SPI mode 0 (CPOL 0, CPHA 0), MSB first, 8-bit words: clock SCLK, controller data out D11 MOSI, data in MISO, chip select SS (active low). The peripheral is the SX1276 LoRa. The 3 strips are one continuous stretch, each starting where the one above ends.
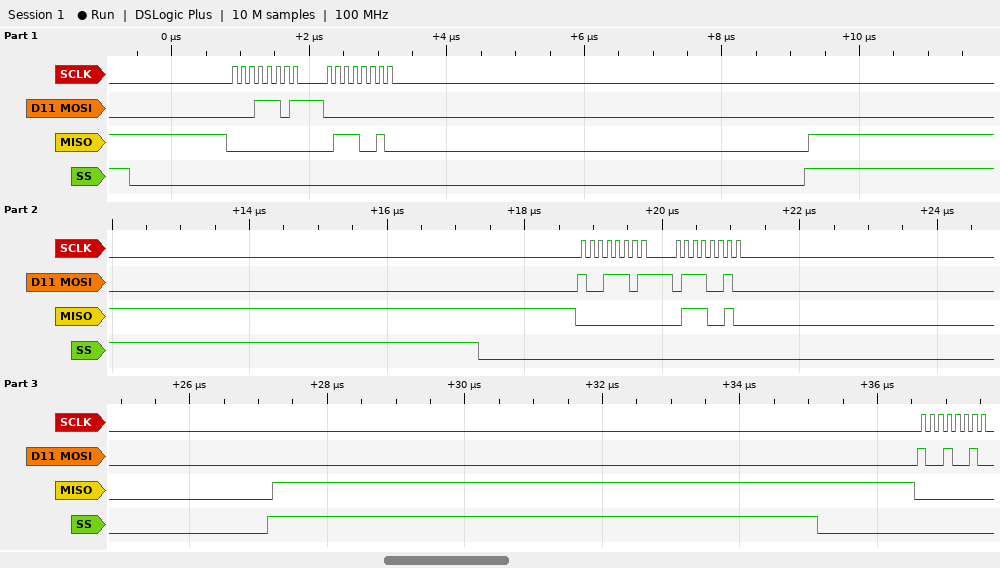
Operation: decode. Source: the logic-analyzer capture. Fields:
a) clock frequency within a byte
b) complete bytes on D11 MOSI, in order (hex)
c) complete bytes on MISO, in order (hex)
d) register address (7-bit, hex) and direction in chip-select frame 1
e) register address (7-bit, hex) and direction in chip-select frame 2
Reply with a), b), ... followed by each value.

a) 8 MHz
b) 1D 00 9D 72 92
c) 00 72 00 72 00
d) 0x1D read
e) 0x1D write
